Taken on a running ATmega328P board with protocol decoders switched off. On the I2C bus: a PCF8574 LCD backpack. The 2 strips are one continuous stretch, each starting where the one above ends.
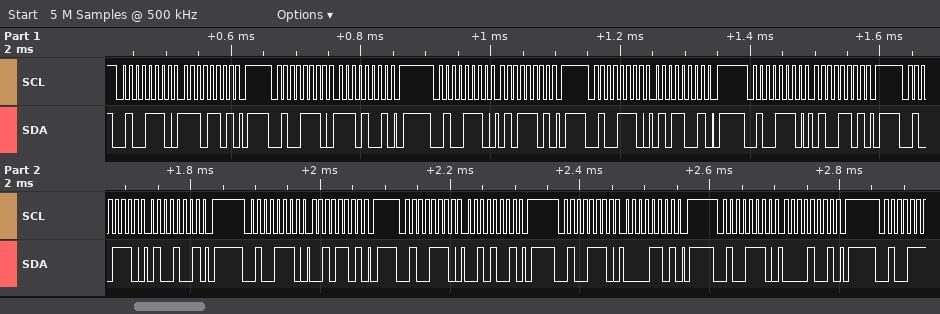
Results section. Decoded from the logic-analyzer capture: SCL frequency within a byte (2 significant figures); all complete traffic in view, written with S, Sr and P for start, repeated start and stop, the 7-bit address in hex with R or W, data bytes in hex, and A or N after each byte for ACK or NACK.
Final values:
100 kHz
S 27W A ED A P S 27W A E9 A P S 27W A 5D A P S 27W A 59 A P S 27W A 4D A P S 27W A 49 A P S 27W A 2D A P S 27W A 29 A P S 27W A 0D A P S 27W A 09 A P
